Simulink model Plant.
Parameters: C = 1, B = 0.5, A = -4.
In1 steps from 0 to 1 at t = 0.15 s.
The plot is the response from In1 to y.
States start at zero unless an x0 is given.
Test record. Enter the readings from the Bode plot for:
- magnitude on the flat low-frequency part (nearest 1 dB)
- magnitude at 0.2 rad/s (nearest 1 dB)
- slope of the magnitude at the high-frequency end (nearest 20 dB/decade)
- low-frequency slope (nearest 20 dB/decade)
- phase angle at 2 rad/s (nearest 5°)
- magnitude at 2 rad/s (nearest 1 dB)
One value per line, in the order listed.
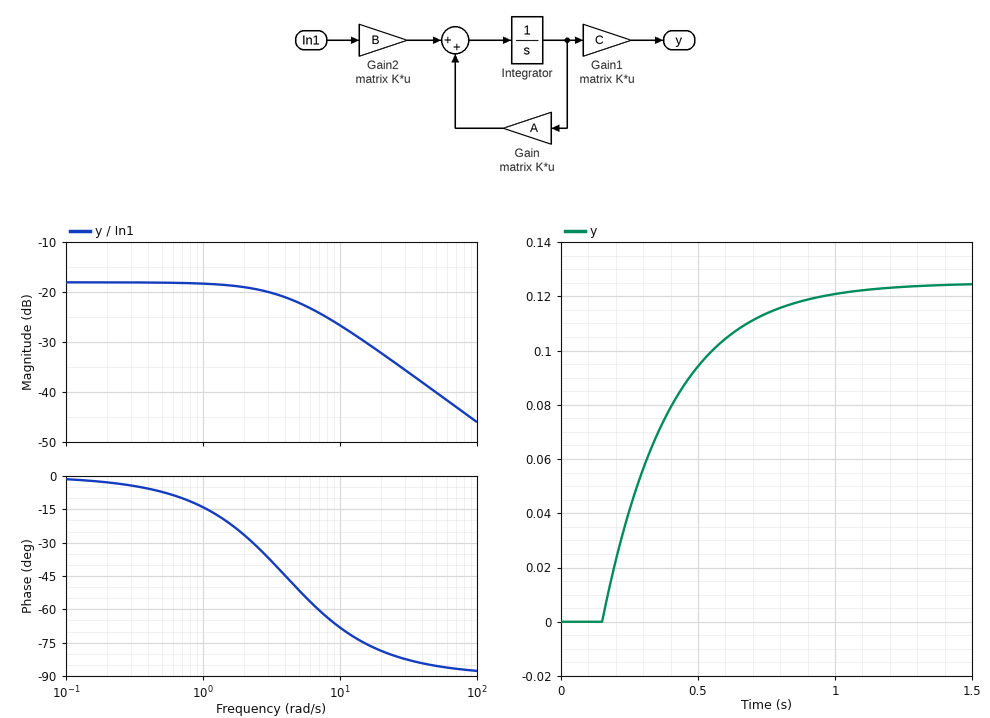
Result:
-18 dB
-18 dB
-20 dB/decade
0 dB/decade
-25°
-19 dB
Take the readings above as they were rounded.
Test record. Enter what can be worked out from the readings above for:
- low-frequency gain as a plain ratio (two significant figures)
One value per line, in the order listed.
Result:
0.13
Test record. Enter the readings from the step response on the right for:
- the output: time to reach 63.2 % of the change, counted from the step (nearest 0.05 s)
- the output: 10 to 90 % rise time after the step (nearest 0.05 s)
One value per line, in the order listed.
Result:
0.25 s
0.55 s
